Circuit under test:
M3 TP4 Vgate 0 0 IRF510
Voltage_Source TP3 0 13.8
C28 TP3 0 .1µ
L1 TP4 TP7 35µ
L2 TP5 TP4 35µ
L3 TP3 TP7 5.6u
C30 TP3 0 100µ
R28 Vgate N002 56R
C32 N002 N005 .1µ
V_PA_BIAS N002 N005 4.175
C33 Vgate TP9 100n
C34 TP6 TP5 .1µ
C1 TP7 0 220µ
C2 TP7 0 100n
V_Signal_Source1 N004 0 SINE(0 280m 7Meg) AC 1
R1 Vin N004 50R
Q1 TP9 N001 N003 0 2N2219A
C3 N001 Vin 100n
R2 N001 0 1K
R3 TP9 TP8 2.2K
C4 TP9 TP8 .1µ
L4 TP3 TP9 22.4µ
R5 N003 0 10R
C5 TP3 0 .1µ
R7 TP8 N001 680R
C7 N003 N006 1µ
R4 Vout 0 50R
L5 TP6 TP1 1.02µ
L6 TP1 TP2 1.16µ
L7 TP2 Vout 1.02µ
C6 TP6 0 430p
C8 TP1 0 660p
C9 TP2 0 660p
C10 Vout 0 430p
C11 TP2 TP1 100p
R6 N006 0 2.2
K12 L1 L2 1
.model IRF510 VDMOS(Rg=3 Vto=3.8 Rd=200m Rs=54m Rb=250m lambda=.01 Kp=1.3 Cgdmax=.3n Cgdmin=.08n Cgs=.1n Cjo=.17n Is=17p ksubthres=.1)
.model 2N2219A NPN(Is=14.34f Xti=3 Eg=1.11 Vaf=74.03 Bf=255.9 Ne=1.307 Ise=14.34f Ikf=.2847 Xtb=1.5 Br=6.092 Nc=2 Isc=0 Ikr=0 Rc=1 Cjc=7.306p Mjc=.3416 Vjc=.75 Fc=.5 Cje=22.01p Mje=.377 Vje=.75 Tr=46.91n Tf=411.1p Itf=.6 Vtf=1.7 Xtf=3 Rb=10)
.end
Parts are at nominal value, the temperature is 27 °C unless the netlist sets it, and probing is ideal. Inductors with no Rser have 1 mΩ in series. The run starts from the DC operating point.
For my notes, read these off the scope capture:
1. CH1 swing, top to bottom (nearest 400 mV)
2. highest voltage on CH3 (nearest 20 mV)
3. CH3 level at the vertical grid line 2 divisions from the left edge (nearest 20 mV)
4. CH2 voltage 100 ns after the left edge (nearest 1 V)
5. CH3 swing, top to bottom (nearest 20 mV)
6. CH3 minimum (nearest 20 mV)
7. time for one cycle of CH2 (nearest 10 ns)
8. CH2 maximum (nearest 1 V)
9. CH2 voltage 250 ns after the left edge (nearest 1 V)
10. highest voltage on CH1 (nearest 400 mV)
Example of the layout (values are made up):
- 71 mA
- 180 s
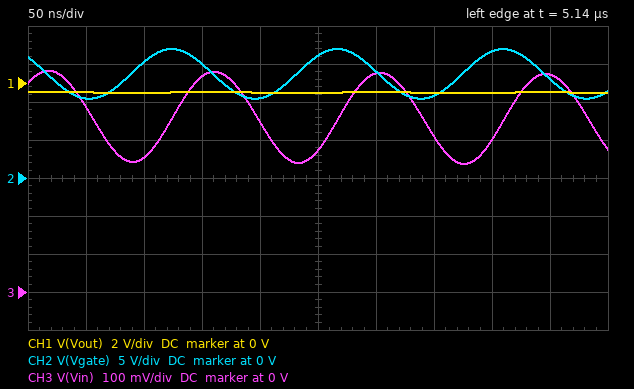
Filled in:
- 0 V
- 580 mV
- 360 mV
- 15 V
- 240 mV
- 340 mV
- 140 ns
- 17 V
- 16 V
- -400 mV
